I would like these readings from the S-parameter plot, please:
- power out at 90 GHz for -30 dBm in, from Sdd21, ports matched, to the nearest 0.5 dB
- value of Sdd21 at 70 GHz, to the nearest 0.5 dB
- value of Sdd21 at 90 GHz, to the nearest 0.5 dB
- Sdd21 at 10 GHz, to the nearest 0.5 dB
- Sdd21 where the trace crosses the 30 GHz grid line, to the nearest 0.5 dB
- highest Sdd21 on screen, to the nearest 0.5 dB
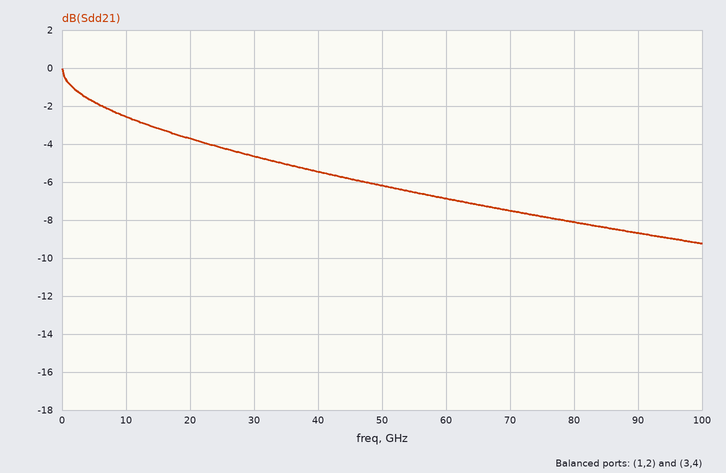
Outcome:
-38.5 dBm
-7.5 dB
-8.5 dB
-2.5 dB
-4.5 dB
0.0 dB
